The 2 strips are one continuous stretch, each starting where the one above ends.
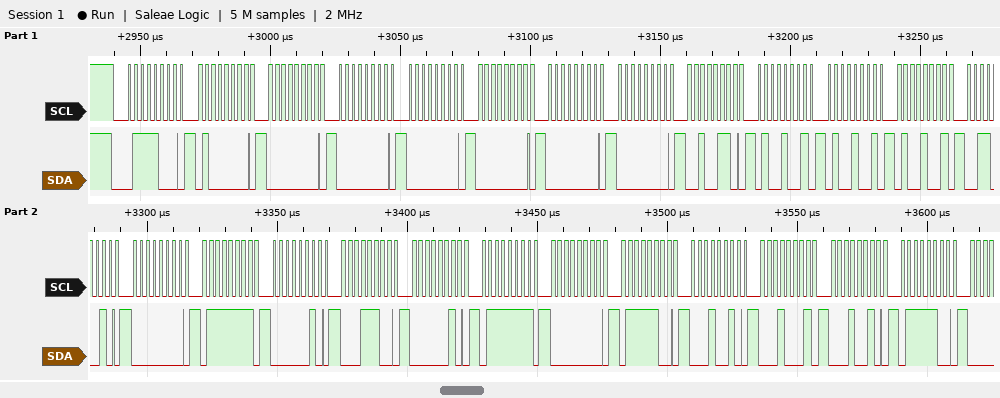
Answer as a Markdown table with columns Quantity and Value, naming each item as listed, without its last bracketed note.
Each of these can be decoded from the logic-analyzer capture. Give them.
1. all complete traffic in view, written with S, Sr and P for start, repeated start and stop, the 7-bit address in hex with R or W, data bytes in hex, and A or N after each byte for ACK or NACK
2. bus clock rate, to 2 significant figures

| Quantity | Value |
|---|---|
| all complete traffic in view, written with S, Sr and P for start, repeated start and stop, the 7-bit address in hex with R or W, data bytes in hex, and A or N after each byte for ACK or NACK | S 3CW A 40 A 00 A 00 A 00 A 00 A 00 A 00 A 26 A 49 A 49 A 49 A 32 A 00 A 7F A 02 A 1C A 02 A 7F A 00 A 7C A 12 A 11 A 12 A 7C A |
| bus clock rate, to 2 significant figures | 400 kHz |
